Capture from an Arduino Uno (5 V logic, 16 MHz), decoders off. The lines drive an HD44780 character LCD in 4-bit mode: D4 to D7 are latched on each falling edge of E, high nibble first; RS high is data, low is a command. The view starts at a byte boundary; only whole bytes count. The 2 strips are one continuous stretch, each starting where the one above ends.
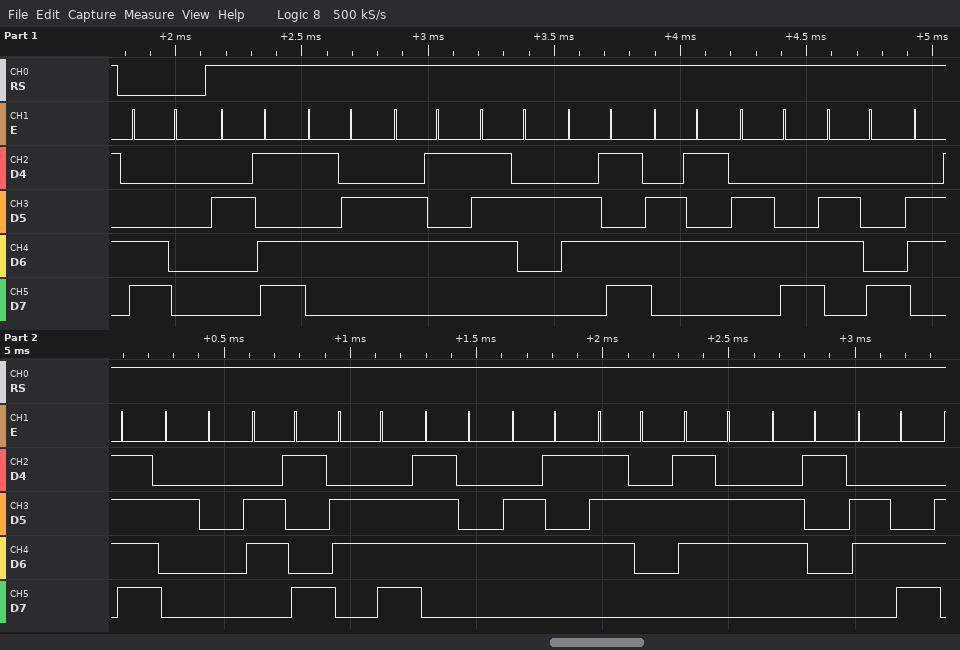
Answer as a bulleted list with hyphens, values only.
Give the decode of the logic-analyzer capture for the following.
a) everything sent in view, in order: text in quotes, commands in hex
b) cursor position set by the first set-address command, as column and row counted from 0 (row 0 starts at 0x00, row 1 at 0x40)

- 0xC0 "-Vermelho interval"
- column 0, row 1
